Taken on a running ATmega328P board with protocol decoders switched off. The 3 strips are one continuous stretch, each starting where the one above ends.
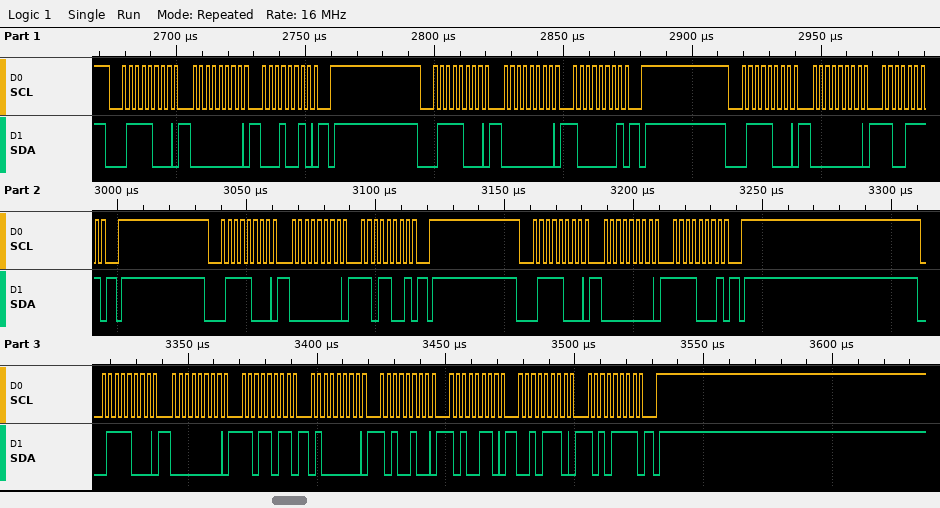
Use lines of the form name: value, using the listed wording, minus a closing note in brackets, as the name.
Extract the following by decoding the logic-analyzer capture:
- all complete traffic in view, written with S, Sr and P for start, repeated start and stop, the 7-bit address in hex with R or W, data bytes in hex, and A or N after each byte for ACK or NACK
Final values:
all complete traffic in view, written with S, Sr and P for start, repeated start and stop, the 7-bit address in hex with R or W, data bytes in hex, and A or N after each byte for ACK or NACK: S 3CW A 00 A 12 A P S 3CW A 00 A 81 A P S 3CW A 00 A CF A P S 3CW A 00 A D9 A P S 3CW A 00 A F1 A P S 3CW A 00 A DB A 40 A A4 A A6 A 2E A AF A P
